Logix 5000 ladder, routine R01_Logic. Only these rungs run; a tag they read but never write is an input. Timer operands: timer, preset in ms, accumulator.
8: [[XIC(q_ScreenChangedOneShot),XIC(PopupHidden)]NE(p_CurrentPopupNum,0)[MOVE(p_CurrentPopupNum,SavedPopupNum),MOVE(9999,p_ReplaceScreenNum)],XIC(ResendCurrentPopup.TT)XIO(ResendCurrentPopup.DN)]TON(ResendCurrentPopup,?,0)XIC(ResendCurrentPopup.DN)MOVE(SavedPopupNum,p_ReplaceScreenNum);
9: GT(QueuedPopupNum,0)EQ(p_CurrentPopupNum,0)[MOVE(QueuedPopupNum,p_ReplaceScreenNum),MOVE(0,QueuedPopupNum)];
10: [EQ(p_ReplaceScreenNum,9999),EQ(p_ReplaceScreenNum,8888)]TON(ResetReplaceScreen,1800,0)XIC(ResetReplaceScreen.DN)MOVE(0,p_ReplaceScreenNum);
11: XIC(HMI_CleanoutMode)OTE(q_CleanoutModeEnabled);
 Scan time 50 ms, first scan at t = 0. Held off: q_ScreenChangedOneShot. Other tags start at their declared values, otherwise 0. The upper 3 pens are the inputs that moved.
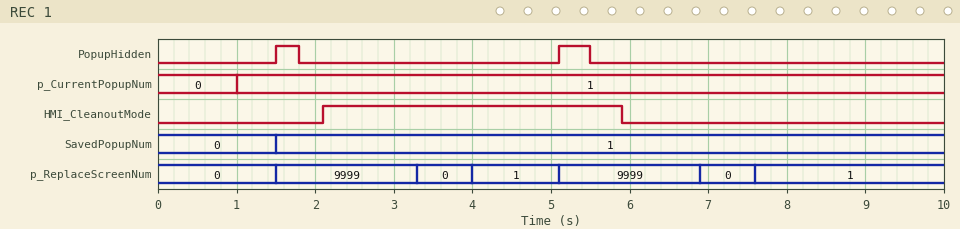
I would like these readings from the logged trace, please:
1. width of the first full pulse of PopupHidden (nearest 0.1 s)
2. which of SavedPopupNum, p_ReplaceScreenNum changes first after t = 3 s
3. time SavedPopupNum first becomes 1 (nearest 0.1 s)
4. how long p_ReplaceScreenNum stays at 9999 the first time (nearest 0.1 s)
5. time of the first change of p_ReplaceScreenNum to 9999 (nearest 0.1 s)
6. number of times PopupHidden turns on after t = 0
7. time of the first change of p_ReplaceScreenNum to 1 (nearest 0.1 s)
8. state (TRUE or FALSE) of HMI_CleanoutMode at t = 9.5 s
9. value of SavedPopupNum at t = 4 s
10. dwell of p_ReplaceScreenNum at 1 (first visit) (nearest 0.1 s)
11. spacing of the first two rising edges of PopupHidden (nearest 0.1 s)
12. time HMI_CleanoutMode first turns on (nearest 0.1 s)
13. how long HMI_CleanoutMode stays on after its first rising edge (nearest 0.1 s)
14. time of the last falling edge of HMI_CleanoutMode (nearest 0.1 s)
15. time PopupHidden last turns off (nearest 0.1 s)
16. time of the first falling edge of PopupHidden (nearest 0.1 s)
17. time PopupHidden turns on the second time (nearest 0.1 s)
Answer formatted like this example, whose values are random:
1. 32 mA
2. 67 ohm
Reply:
1. 0.3 s
2. p_ReplaceScreenNum
3. 1.5 s
4. 1.8 s
5. 1.5 s
6. 2
7. 4.0 s
8. FALSE
9. 1
10. 1.1 s
11. 3.6 s
12. 2.1 s
13. 3.8 s
14. 5.9 s
15. 5.5 s
16. 1.8 s
17. 5.1 s
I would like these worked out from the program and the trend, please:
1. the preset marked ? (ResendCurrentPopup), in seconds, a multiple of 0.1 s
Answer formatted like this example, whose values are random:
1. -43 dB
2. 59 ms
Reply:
1. 2.5 s
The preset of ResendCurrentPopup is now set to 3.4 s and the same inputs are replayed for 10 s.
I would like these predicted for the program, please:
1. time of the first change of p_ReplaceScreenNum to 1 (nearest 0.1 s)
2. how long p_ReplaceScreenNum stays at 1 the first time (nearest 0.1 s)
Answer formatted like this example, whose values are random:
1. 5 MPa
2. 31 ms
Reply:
1. 4.9 s
2. 0.2 s
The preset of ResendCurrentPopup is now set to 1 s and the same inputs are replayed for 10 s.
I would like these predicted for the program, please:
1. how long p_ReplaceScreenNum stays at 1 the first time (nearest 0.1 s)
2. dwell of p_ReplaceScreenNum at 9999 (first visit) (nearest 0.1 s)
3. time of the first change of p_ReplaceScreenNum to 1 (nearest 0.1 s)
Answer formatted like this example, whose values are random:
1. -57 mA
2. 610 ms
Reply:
1. 2.6 s
2. 1.0 s
3. 2.5 s
